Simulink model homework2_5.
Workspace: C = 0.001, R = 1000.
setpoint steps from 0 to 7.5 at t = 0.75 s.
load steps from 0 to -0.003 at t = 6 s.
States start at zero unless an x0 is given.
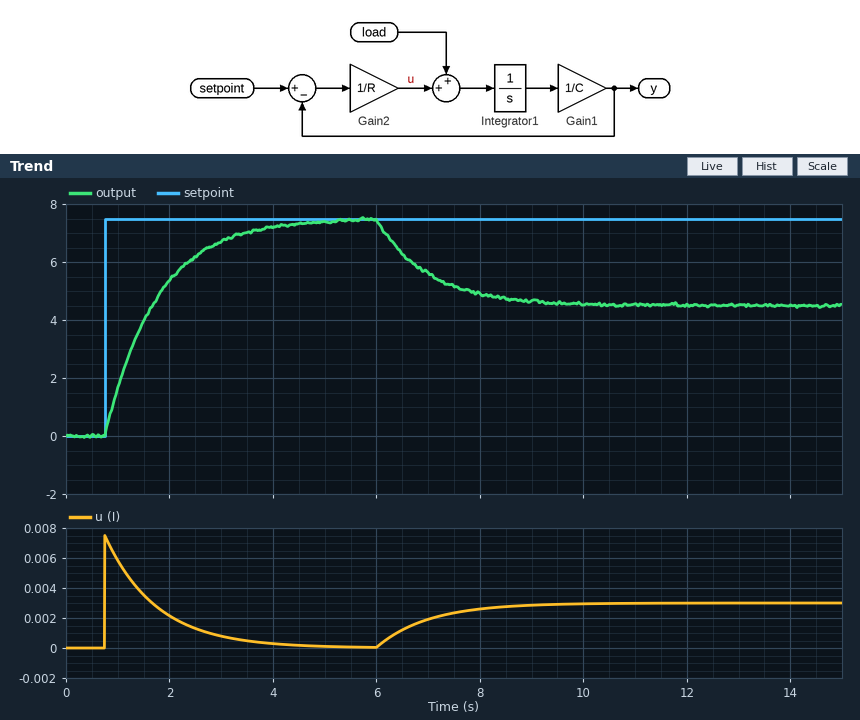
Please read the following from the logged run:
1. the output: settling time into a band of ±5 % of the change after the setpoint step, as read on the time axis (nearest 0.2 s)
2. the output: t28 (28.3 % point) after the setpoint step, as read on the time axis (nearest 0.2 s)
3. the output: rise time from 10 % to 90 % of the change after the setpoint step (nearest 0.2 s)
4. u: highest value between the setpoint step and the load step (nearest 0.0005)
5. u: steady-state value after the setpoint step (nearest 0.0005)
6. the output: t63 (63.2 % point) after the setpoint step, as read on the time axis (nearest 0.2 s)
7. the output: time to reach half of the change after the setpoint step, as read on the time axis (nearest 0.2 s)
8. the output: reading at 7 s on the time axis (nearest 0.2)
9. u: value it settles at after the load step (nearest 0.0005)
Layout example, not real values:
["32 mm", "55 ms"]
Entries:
["3.8 s", "1.0 s", "2.2 s", "0.0075", "0.0000", "1.8 s", "1.4 s", "5.6", "0.0030"]
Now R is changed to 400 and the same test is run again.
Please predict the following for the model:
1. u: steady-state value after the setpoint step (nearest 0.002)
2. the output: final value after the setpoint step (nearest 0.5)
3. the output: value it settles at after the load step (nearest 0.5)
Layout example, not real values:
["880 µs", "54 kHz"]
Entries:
["0.000", "7.5", "6.5"]
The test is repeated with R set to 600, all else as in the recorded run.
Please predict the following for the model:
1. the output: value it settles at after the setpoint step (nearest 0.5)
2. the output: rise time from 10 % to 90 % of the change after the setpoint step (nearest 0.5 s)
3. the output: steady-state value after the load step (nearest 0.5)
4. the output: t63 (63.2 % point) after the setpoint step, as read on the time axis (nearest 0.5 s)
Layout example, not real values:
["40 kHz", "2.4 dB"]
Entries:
["7.5", "1.5 s", "5.5", "1.5 s"]
